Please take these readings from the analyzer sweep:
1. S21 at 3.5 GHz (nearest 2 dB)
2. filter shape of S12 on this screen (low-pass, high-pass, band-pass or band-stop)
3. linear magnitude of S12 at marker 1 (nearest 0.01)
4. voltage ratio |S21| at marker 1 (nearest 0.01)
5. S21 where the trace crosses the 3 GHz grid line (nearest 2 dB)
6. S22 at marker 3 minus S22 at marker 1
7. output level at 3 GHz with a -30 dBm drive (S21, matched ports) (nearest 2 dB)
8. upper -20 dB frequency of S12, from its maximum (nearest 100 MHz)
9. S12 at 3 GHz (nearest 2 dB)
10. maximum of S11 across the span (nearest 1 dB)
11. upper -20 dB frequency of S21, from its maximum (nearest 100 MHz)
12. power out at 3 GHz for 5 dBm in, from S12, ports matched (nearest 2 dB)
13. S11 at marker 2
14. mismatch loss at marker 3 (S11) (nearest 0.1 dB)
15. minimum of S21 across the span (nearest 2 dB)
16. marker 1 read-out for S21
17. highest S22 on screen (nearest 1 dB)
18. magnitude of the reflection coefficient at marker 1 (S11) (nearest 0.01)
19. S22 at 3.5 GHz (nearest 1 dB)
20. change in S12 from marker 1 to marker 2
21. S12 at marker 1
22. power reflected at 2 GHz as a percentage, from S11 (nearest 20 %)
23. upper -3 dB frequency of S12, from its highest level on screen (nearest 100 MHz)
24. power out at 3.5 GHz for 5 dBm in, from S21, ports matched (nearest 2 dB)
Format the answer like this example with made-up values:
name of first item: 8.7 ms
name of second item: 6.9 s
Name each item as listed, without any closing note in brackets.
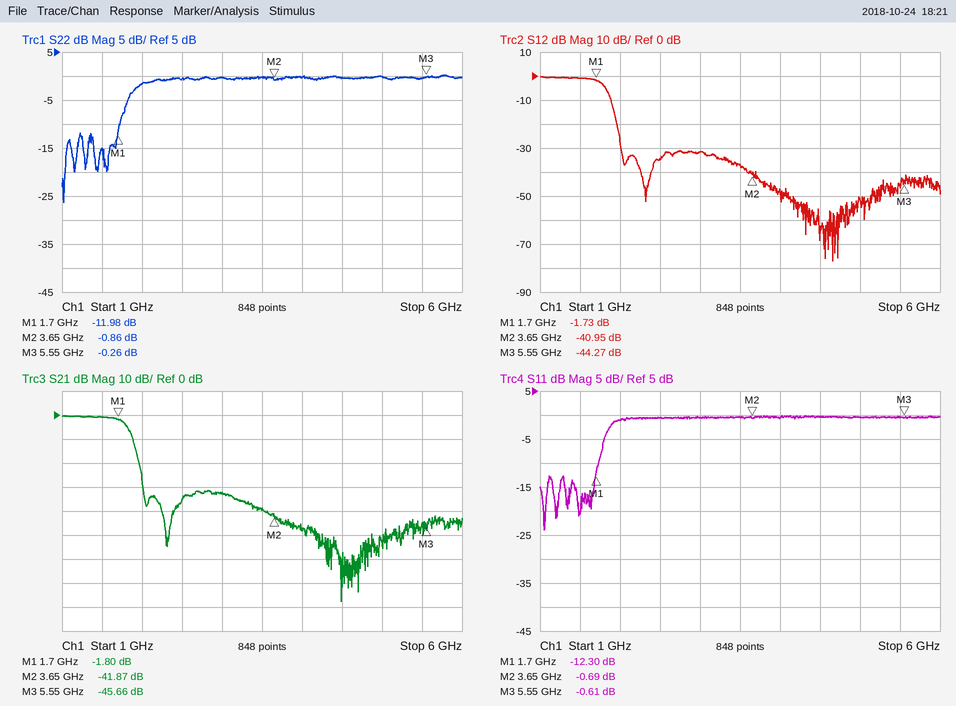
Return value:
S21 at 3.5 GHz: -40 dB
filter shape of S12 on this screen: low-pass
linear magnitude of S12 at marker 1: 0.82
voltage ratio |S21| at marker 1: 0.81
S21 where the trace crosses the 3 GHz grid line: -32 dB
S22 at marker 3 minus S22 at marker 1: 11.72 dB
output level at 3 GHz with a -30 dBm drive (S21, matched ports): -62 dBm
upper -20 dB frequency of S12, from its maximum: 2.0 GHz
S12 at 3 GHz: -32 dB
maximum of S11 across the span: 0 dB
upper -20 dB frequency of S21, from its maximum: 2.0 GHz
power out at 3 GHz for 5 dBm in, from S12, ports matched: -26 dBm
S11 at marker 2: -0.69 dB
mismatch loss at marker 3 (S11): 8.8 dB
minimum of S21 across the span: -78 dB
marker 1 read-out for S21: -1.80 dB
highest S22 on screen: 0 dB
magnitude of the reflection coefficient at marker 1 (S11): 0.24
S22 at 3.5 GHz: 0 dB
change in S12 from marker 1 to marker 2: -39.22 dB
S12 at marker 1: -1.73 dB
power reflected at 2 GHz as a percentage, from S11: 80 %
upper -3 dB frequency of S12, from its highest level on screen: 1.8 GHz
power out at 3.5 GHz for 5 dBm in, from S21, ports matched: -34 dBm
